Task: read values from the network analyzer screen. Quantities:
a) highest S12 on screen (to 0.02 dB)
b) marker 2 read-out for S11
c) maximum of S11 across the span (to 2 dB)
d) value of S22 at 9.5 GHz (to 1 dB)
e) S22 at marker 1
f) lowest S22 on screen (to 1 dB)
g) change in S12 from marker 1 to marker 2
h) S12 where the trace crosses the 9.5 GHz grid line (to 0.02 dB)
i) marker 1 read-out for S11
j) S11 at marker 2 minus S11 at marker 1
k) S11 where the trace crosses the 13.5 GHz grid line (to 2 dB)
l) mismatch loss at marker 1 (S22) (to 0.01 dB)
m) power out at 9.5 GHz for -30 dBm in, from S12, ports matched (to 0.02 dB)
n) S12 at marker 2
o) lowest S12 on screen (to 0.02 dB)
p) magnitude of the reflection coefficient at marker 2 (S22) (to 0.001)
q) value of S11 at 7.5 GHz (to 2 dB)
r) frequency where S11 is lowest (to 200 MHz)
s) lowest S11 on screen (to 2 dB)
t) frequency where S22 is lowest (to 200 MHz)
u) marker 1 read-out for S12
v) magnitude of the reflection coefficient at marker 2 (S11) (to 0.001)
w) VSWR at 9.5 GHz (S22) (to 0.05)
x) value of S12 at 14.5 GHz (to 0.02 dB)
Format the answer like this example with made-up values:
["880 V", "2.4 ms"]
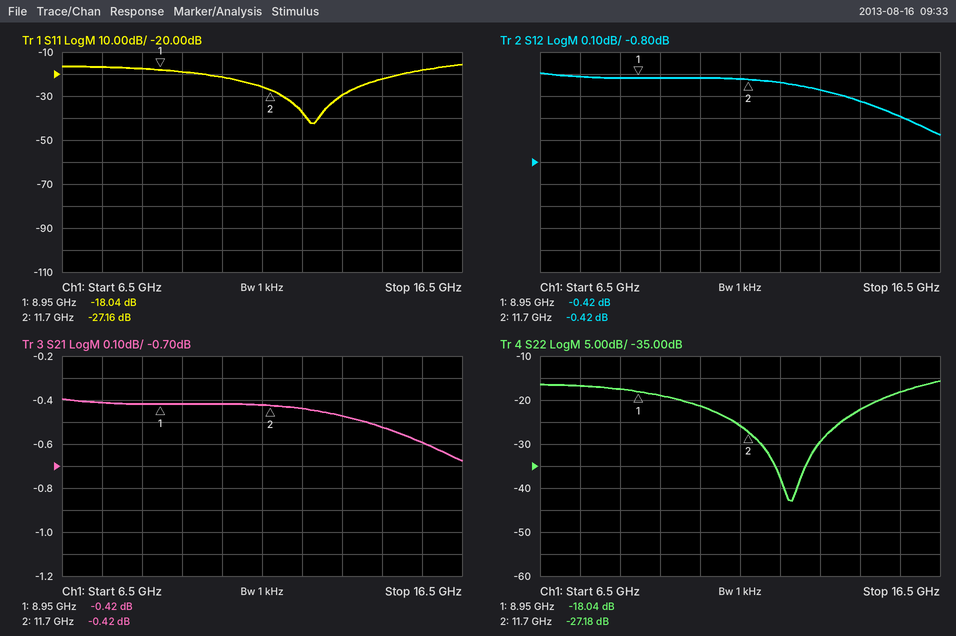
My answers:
["-0.40 dB", "-27.16 dB", "-16 dB", "-19 dB", "-18.04 dB", "-43 dB", "0.00 dB", "-0.42 dB", "-18.04 dB", "-9.12 dB", "-30 dB", "0.07 dB", "-30.42 dBm", "-0.42 dB", "-0.68 dB", "0.044", "-16 dB", "12.8 GHz", "-42 dB", "12.8 GHz", "-0.42 dB", "0.044", "1.25", "-0.52 dB"]
